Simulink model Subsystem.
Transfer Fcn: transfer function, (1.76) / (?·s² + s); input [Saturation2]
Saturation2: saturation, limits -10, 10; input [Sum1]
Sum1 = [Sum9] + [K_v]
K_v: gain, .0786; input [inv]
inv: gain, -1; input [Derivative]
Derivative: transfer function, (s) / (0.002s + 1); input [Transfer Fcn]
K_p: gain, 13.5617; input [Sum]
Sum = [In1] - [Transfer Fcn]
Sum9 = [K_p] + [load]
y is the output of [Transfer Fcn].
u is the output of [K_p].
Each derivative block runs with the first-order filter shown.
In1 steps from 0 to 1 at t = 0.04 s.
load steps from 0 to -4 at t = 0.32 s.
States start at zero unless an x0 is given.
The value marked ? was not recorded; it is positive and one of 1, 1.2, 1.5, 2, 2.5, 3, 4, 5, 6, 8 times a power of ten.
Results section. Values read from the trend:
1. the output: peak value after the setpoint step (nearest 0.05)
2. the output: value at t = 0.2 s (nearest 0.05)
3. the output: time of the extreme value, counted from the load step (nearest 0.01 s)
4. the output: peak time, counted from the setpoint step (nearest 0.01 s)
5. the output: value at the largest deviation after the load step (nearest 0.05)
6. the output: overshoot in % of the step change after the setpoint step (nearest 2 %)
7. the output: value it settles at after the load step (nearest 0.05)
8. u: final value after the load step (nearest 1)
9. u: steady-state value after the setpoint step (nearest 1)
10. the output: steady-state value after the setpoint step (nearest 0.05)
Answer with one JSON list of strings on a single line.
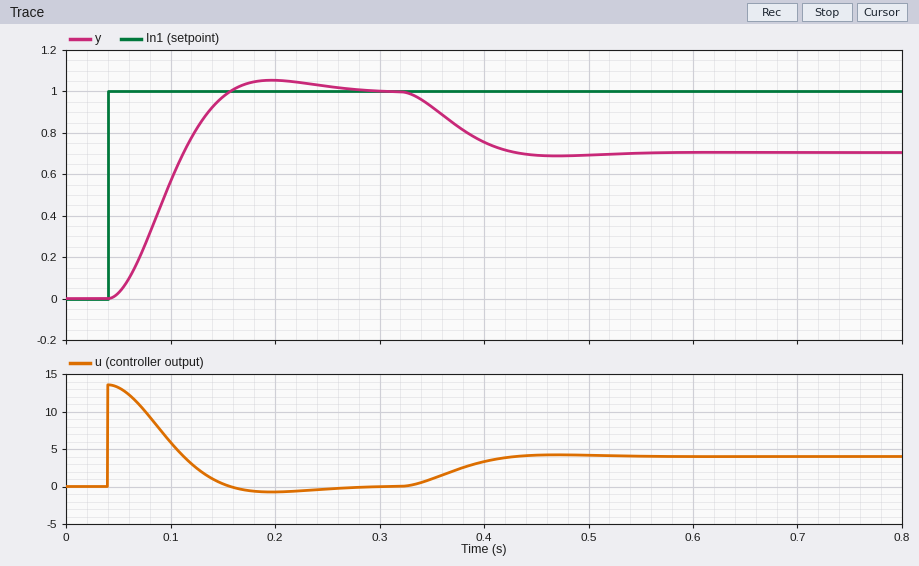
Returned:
["1.05", "1.05", "0.15 s", "0.16 s", "0.70", "6 %", "0.70", "4", "0", "1.00"]
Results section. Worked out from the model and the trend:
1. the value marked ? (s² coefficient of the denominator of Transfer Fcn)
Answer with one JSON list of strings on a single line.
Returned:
["0.03"]
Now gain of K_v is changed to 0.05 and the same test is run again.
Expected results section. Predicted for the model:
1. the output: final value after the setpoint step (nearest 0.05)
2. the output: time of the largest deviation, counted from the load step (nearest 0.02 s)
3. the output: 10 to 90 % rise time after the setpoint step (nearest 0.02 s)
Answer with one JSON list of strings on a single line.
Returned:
["1.00", "0.14 s", "0.08 s"]
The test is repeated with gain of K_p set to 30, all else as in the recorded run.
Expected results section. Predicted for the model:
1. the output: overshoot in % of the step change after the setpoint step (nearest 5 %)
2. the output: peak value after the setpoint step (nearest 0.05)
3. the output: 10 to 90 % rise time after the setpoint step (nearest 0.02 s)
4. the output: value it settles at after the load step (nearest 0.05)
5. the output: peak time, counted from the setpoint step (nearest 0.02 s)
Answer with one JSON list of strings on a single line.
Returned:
["15 %", "1.15", "0.06 s", "0.85", "0.12 s"]
